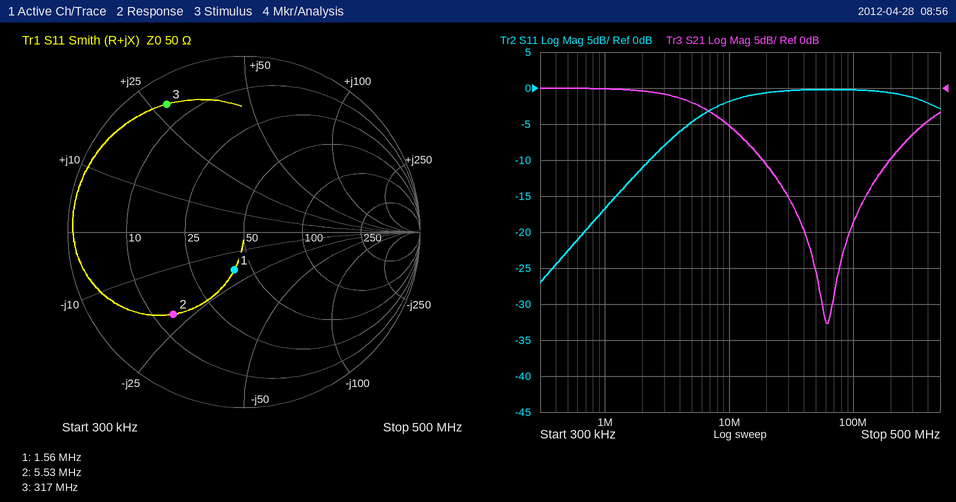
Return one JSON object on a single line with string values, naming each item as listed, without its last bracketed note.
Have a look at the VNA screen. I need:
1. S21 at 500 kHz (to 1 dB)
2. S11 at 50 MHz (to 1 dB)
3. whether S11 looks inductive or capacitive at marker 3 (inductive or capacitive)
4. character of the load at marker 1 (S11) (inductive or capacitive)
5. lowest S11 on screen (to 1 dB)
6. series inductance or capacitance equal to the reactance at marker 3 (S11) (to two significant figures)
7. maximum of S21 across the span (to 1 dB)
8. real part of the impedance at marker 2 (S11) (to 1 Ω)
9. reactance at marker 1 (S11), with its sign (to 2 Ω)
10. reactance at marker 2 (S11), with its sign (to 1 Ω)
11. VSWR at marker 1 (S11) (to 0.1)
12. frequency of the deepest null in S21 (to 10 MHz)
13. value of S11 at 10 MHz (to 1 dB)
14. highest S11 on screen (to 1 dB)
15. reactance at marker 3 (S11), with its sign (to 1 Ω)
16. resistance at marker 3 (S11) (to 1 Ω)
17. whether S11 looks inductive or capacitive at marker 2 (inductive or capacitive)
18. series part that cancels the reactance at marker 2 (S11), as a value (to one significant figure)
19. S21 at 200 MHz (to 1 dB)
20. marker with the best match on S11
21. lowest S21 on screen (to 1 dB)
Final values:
{"S21 at 500 kHz": "0 dB", "S11 at 50 MHz": "0 dB", "whether S11 looks inductive or capacitive at marker 3": "inductive", "character of the load at marker 1 (S11)": "capacitive", "lowest S11 on screen": "-27 dB", "series inductance or capacitance equal to the reactance at marker 3 (S11)": "14 nH", "maximum of S21 across the span": "0 dB", "real part of the impedance at marker 2 (S11)": "14 Ω", "reactance at marker 1 (S11), with its sign": "-18 Ω", "reactance at marker 2 (S11), with its sign": "-21 Ω", "VSWR at marker 1 (S11)": "1.6", "frequency of the deepest null in S21": "60 MHz", "value of S11 at 10 MHz": "-2 dB", "highest S11 on screen": "0 dB", "reactance at marker 3 (S11), with its sign": "+28 Ω", "resistance at marker 3 (S11)": "5 Ω", "whether S11 looks inductive or capacitive at marker 2": "capacitive", "series part that cancels the reactance at marker 2 (S11), as a value": "600 nH", "S21 at 200 MHz": "-10 dB", "marker with the best match on S11": "marker 1", "lowest S21 on screen": "-33 dB"}
